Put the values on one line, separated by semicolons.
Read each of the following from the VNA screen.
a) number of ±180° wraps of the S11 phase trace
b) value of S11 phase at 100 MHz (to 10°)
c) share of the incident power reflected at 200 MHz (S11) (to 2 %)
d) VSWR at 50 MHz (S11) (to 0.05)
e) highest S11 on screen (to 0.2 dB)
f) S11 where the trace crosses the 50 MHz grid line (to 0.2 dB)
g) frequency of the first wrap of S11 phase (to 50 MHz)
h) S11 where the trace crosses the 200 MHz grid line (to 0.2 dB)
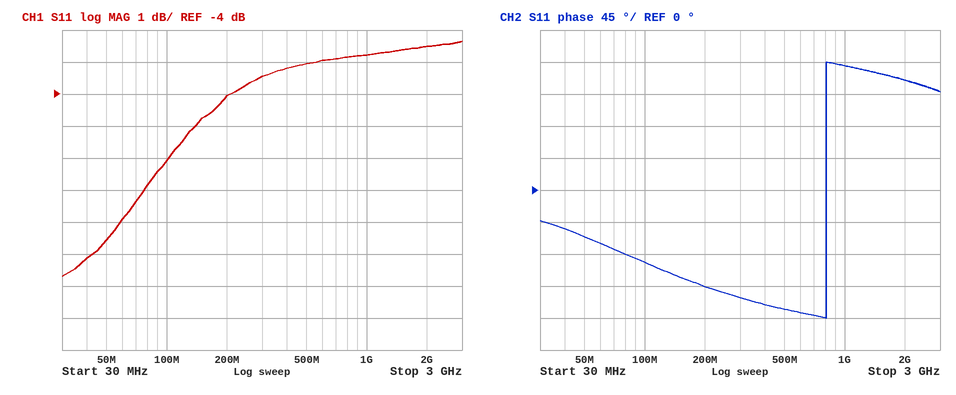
1; -100°; 40 %; 2.20; -2.4 dB; -8.6 dB; 800 MHz; -4.0 dB
